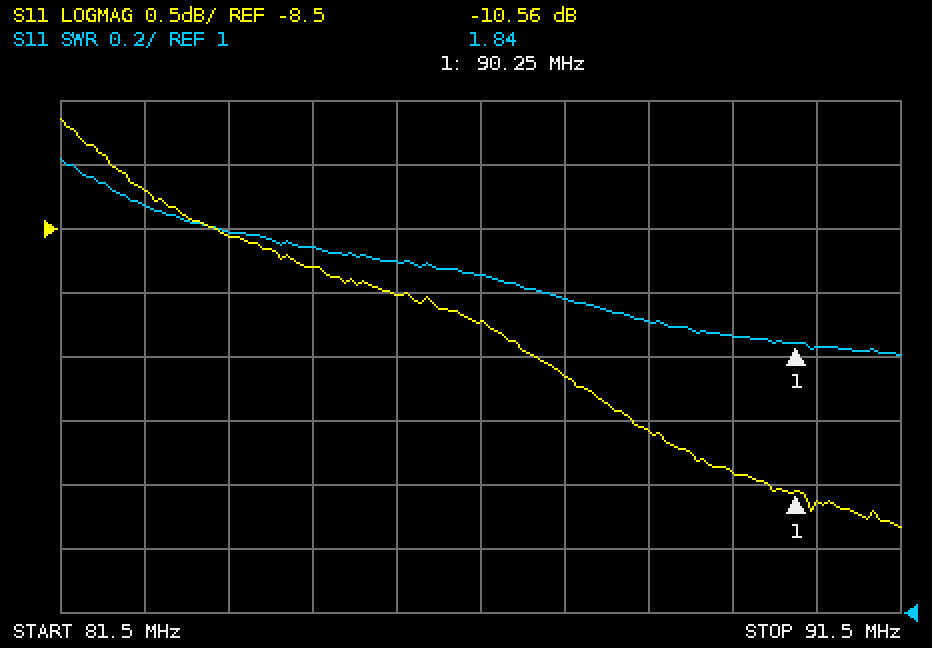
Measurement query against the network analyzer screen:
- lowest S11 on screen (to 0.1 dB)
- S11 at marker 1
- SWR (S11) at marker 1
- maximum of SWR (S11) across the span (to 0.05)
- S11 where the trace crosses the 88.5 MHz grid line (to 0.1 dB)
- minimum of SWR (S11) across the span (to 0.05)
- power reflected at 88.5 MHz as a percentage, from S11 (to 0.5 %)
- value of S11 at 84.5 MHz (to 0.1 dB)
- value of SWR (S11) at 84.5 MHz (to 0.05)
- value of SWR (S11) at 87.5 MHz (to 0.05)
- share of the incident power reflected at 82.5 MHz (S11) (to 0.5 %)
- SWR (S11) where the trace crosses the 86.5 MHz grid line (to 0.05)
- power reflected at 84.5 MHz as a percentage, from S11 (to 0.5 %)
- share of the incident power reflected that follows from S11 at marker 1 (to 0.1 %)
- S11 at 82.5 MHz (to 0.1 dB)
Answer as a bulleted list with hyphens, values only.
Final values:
- -10.8 dB
- -10.56 dB
- 1.84
- 2.40
- -10.1 dB
- 1.80
- 10.0 %
- -8.8 dB
- 2.15
- 2.00
- 15.0 %
- 2.05
- 13.0 %
- 8.8 %
- -8.2 dB
